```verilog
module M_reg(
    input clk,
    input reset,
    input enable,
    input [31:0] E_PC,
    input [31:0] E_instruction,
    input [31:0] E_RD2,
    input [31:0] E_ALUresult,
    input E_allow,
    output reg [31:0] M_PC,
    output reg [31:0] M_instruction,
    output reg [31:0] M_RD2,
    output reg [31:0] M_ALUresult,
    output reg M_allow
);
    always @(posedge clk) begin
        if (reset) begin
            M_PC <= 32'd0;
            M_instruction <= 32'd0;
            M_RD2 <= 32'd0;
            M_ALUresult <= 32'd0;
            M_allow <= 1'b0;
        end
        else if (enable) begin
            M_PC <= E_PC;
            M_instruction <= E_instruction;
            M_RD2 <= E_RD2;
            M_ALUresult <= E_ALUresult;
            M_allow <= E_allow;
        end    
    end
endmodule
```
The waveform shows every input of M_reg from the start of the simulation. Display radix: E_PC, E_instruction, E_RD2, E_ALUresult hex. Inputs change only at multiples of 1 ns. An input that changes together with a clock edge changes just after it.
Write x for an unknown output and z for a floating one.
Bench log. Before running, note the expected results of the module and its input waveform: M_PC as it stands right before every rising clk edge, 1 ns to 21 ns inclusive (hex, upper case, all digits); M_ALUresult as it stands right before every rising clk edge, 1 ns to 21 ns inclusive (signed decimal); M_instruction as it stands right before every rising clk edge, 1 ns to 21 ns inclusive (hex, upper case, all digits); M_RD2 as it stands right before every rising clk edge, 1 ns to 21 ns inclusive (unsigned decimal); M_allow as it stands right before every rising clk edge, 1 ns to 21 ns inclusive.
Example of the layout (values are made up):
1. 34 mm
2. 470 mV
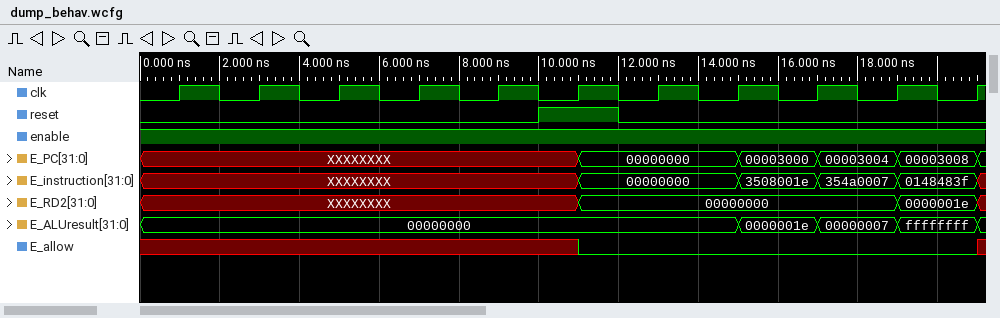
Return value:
1. x, x, x, x, x, x, 00000000, 00000000, 00000000, 00003000, 00003004
2. x, 0, 0, 0, 0, 0, 0, 0, 0, 30, 7
3. x, x, x, x, x, x, 00000000, 00000000, 00000000, 3508001E, 354A0007
4. x, x, x, x, x, x, 0, 0, 0, 0, 0
5. x x x x x x 0 0 0 0 0
